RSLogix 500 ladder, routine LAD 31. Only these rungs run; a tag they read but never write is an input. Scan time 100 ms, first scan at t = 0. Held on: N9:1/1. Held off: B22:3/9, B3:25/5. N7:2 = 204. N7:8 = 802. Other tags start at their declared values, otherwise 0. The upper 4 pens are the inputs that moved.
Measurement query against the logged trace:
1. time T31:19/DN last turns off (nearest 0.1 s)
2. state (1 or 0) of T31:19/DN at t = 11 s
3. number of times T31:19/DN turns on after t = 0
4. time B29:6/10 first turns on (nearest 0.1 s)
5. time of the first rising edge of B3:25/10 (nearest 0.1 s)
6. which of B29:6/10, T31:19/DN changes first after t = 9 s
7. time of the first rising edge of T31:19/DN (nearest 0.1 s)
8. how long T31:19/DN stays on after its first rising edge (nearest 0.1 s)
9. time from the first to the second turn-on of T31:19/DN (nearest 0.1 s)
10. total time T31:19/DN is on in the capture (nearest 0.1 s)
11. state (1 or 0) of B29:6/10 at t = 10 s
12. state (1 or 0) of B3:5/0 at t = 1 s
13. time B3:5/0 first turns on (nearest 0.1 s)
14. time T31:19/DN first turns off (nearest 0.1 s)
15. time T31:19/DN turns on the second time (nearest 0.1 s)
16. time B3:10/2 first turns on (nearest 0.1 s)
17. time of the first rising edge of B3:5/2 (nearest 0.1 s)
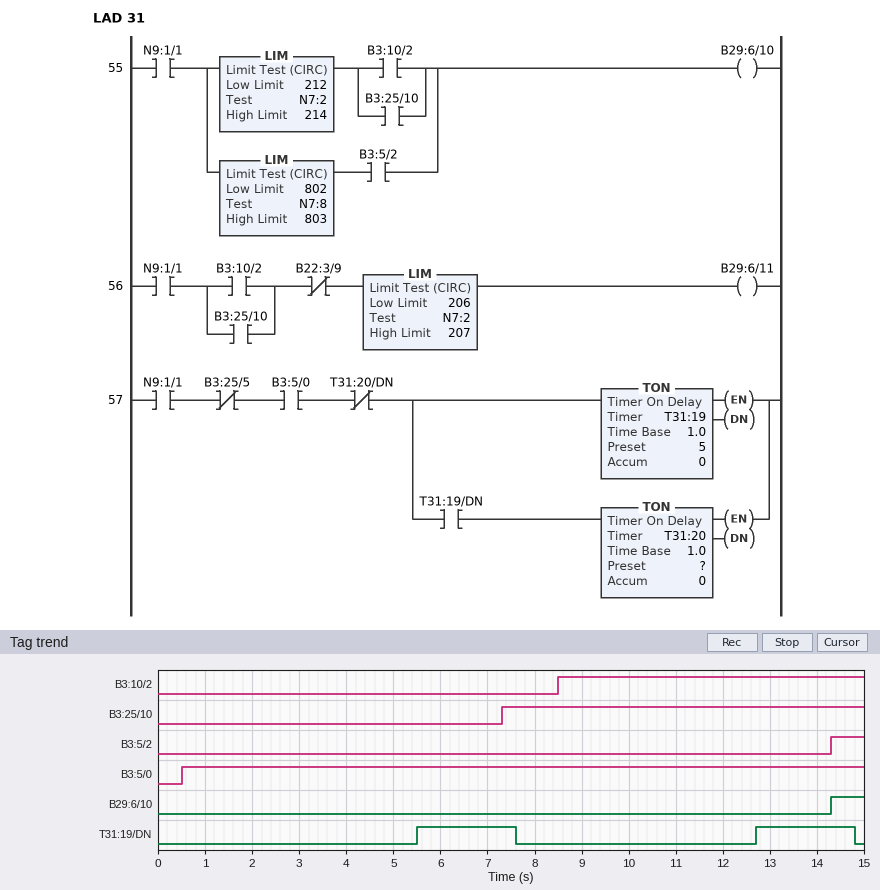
14.8 s
0
2
14.3 s
7.3 s
T31:19/DN
5.5 s
2.1 s
7.2 s
4.2 s
0
1
0.5 s
7.6 s
12.7 s
8.5 s
14.3 s
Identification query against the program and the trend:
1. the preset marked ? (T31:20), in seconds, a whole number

2 s
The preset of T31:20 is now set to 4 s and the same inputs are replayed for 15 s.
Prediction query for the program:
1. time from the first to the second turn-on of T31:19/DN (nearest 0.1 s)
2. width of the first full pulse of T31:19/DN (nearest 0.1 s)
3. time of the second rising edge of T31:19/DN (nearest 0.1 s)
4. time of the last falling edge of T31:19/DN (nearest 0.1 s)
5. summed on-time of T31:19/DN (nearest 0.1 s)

9.2 s
4.1 s
14.7 s
9.6 s
4.4 s
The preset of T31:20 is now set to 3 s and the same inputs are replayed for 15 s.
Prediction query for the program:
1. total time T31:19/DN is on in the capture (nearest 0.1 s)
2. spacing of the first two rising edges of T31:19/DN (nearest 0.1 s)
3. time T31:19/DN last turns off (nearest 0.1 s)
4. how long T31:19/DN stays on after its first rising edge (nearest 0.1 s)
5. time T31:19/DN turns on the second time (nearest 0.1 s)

4.4 s
8.2 s
8.6 s
3.1 s
13.7 s
